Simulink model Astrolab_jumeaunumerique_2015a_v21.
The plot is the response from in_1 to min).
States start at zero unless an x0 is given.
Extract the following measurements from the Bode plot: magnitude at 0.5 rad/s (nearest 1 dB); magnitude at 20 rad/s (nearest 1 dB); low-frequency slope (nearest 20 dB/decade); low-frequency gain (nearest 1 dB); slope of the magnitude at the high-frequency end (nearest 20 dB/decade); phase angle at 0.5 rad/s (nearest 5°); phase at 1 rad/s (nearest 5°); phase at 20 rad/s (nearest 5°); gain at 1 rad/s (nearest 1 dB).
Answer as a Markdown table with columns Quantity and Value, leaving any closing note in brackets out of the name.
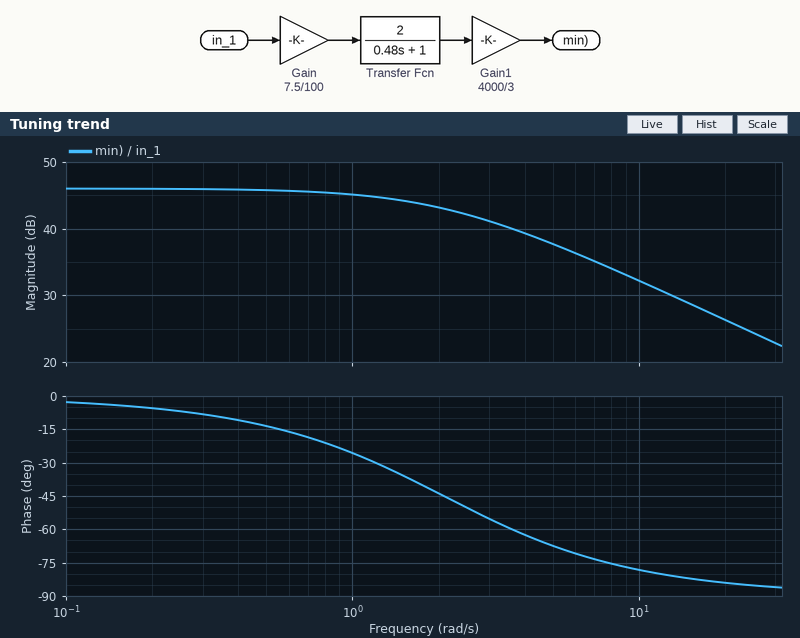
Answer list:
| Quantity | Value |
|---|---|
| magnitude at 0.5 rad/s | 46 dB |
| magnitude at 20 rad/s | 26 dB |
| low-frequency slope | 0 dB/decade |
| low-frequency gain | 46 dB |
| slope of the magnitude at the high-frequency end | -20 dB/decade |
| phase angle at 0.5 rad/s | -15° |
| phase at 1 rad/s | -25° |
| phase at 20 rad/s | -85° |
| gain at 1 rad/s | 45 dB |
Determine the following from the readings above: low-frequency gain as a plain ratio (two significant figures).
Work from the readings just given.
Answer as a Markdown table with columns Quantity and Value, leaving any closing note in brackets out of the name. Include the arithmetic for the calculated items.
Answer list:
| Quantity | Value |
|---|---|
| low-frequency gain as a plain ratio | 10^(46 / 20) = 200 |
